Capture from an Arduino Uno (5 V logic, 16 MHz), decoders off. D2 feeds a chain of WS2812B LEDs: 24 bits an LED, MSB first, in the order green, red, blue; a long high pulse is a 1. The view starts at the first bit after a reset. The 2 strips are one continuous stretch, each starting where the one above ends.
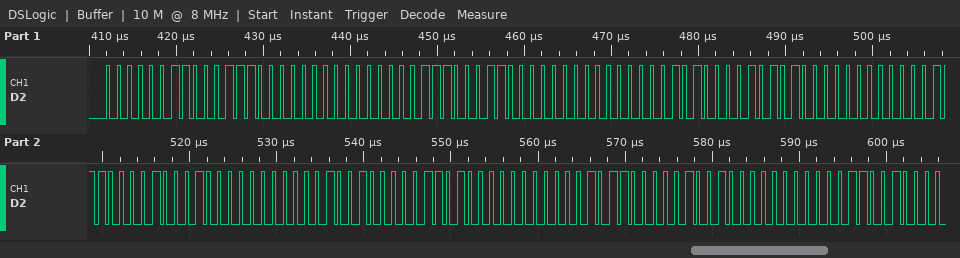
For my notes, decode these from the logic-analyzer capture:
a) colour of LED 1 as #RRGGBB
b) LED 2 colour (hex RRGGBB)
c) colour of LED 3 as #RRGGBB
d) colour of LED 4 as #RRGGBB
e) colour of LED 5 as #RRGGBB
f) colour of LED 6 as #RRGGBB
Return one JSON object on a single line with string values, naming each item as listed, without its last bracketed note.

{"colour of LED 1 as #RRGGBB": "#1C0300", "LED 2 colour": "#180700", "colour of LED 3 as #RRGGBB": "#150A00", "colour of LED 4 as #RRGGBB": "#110E00", "colour of LED 5 as #RRGGBB": "#0D1200", "colour of LED 6 as #RRGGBB": "#091600"}
